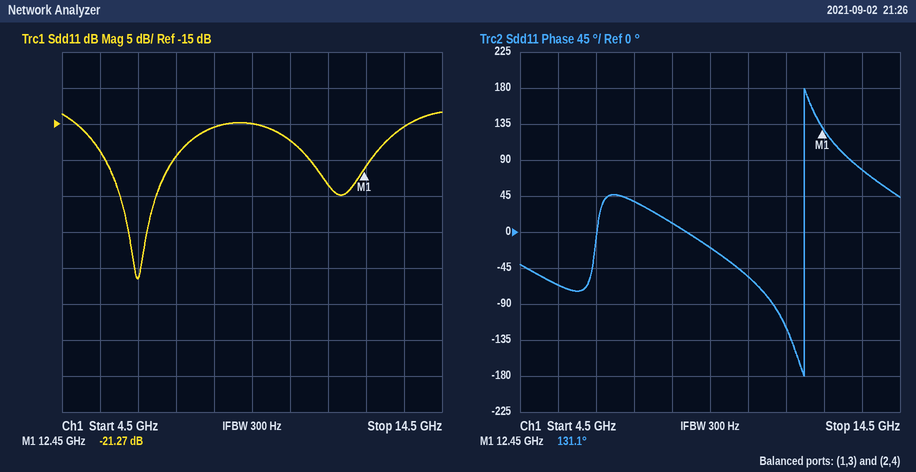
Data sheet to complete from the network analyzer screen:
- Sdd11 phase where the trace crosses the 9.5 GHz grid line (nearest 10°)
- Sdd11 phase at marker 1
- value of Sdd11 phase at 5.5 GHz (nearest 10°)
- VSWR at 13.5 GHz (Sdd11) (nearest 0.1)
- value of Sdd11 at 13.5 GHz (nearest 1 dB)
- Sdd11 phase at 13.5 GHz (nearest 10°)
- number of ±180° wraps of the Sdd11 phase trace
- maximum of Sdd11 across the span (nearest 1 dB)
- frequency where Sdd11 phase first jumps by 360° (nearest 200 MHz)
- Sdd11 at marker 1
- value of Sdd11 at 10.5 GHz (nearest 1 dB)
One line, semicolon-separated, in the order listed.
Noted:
-20°; 131.1°; -70°; 1.4; -15 dB; 80°; 1; -13 dB; 12.0 GHz; -21.27 dB; -17 dB
